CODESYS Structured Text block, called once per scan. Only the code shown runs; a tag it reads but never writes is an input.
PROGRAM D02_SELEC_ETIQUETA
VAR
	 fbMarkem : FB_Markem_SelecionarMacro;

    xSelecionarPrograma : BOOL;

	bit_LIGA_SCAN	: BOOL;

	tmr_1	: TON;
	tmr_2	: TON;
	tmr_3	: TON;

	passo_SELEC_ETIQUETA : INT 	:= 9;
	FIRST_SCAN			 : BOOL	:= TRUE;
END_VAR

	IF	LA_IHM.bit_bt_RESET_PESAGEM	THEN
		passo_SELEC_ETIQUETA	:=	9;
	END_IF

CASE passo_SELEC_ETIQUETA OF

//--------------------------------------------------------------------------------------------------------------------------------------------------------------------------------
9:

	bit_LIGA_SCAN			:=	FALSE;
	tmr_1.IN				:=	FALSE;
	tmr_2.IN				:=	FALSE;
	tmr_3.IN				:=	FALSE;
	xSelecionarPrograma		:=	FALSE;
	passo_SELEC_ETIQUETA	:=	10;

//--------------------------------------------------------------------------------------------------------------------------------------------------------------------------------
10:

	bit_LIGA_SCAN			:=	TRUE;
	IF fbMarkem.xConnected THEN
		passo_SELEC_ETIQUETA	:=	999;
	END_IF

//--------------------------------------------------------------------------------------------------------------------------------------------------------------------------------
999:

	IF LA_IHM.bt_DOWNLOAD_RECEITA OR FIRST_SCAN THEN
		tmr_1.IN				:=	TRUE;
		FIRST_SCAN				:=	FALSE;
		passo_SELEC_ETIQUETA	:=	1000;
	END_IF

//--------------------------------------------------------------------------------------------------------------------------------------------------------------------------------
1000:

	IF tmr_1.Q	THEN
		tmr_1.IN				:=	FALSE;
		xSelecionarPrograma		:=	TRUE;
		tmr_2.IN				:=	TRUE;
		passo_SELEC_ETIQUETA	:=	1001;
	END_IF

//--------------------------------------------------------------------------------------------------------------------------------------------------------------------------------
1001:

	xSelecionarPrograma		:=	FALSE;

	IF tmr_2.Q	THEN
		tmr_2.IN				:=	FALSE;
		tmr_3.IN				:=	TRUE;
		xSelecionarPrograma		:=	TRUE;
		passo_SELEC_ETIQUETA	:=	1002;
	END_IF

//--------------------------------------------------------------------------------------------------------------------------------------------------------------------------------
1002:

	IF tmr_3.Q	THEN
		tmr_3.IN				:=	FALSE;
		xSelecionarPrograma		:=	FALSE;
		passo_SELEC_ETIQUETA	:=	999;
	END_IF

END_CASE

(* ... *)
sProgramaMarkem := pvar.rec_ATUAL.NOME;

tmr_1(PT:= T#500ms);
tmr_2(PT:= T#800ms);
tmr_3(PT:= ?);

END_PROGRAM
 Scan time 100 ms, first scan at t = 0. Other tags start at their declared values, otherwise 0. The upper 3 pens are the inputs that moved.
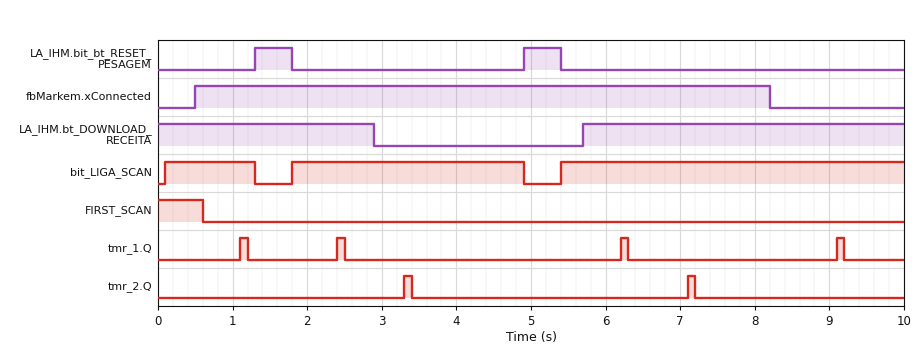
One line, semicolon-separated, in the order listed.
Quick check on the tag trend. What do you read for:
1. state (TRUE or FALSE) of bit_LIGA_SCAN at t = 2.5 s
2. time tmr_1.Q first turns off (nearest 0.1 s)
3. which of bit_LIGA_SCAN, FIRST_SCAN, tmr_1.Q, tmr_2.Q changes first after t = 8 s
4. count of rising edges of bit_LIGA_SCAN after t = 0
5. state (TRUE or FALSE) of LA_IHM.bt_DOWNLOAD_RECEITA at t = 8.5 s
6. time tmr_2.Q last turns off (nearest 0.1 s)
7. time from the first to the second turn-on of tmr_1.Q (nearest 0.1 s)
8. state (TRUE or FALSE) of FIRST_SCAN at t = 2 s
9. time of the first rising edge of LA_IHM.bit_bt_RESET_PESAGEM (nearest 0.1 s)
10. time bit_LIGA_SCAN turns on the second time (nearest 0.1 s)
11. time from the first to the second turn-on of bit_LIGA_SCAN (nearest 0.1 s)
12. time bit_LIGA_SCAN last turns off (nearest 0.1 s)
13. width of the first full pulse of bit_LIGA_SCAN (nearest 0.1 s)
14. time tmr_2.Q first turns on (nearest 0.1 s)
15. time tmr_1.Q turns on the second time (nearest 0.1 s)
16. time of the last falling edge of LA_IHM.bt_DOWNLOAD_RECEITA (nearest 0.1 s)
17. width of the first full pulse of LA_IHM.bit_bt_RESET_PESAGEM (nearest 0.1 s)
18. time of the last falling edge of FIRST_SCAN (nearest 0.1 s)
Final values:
TRUE; 1.2 s; tmr_1.Q; 3; TRUE; 7.2 s; 1.3 s; FALSE; 1.3 s; 1.8 s; 1.7 s; 4.9 s; 1.2 s; 3.3 s; 2.4 s; 2.9 s; 0.5 s; 0.6 s
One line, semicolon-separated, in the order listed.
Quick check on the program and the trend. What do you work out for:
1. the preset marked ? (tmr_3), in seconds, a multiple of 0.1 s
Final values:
1.2 s
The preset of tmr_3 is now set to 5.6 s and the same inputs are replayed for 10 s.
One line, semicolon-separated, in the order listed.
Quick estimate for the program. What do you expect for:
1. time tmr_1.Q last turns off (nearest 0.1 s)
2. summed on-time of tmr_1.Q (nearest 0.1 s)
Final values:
6.3 s; 0.3 s
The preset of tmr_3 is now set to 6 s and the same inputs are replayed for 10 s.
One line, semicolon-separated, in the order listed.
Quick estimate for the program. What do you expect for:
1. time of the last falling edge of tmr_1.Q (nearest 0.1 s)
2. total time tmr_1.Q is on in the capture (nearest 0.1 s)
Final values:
6.3 s; 0.3 s
